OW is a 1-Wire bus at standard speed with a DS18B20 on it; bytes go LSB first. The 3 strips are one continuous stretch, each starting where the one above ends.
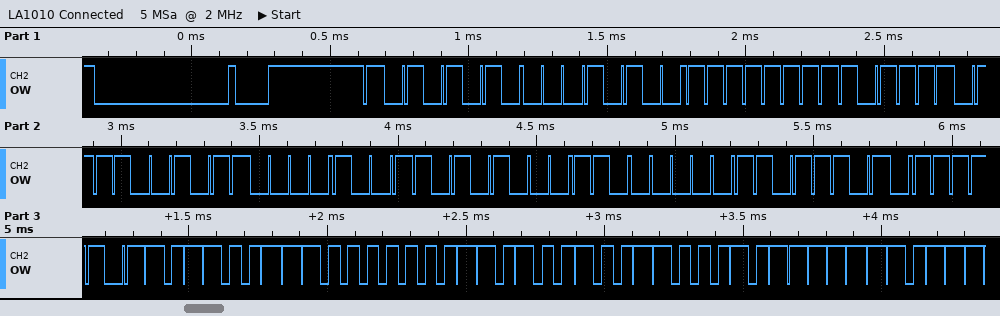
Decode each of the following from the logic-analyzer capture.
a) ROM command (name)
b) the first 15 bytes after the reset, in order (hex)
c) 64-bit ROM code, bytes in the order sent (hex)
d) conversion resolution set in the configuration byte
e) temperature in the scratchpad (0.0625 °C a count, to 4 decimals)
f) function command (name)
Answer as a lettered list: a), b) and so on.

a) Match ROM
b) 55 28 FF BD D3 90 15 03 BB BE CD 01 4B 46 7F
c) 28 FF BD D3 90 15 03 BB
d) 12 bits
e) 28.8125 °C
f) Read Scratchpad
